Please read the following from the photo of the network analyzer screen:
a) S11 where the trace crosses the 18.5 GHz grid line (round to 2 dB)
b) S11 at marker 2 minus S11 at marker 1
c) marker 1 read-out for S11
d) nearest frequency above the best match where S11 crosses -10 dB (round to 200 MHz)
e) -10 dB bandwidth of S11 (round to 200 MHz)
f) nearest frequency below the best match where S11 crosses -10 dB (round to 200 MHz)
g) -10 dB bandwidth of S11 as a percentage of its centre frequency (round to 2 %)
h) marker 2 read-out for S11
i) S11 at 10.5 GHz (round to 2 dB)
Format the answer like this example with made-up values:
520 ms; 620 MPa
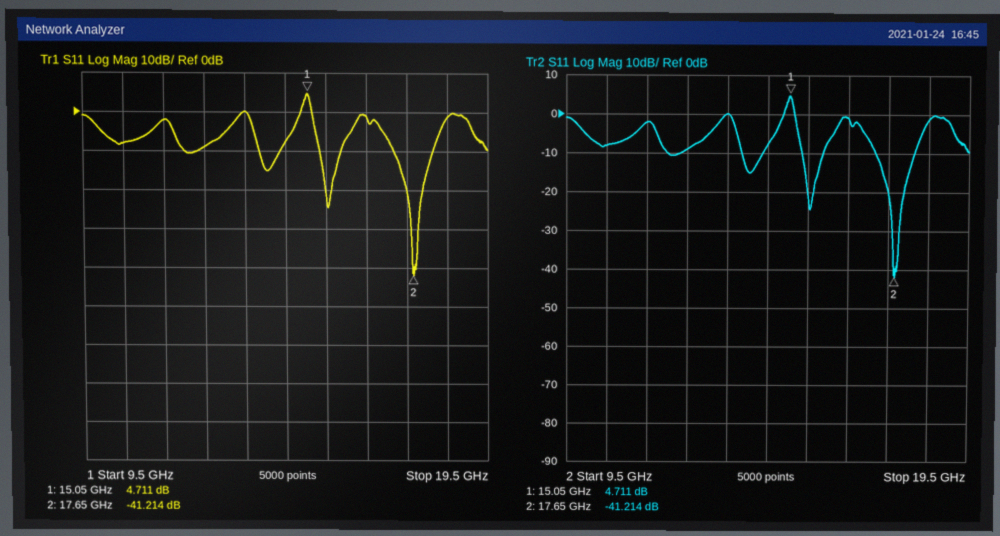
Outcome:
-2 dB; -45.925 dB; 4.711 dB; 18.2 GHz; 1.0 GHz; 17.2 GHz; 6 %; -41.214 dB; -8 dB
